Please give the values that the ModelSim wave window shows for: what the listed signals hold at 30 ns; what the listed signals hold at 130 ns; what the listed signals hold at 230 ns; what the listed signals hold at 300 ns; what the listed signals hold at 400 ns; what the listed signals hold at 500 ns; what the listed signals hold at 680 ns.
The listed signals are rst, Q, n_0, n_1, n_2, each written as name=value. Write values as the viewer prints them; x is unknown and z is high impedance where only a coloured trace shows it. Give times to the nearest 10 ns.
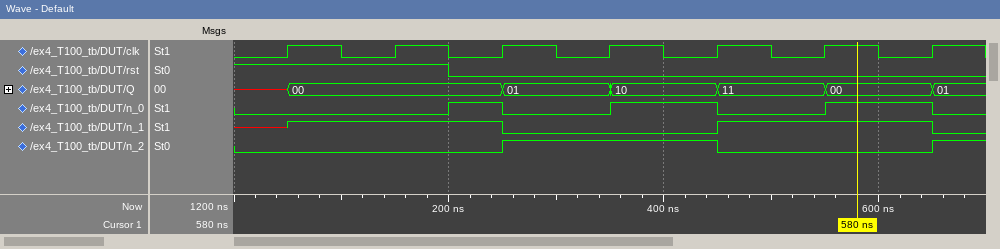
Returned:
rst=1, Q=x, n_0=0, n_1=x, n_2=0
rst=1, Q=00, n_0=0, n_1=1, n_2=0
rst=0, Q=00, n_0=1, n_1=1, n_2=0
rst=0, Q=01, n_0=0, n_1=0, n_2=1
rst=0, Q=10, n_0=1, n_1=0, n_2=1
rst=0, Q=11, n_0=0, n_1=1, n_2=0
rst=0, Q=01, n_0=0, n_1=0, n_2=1
